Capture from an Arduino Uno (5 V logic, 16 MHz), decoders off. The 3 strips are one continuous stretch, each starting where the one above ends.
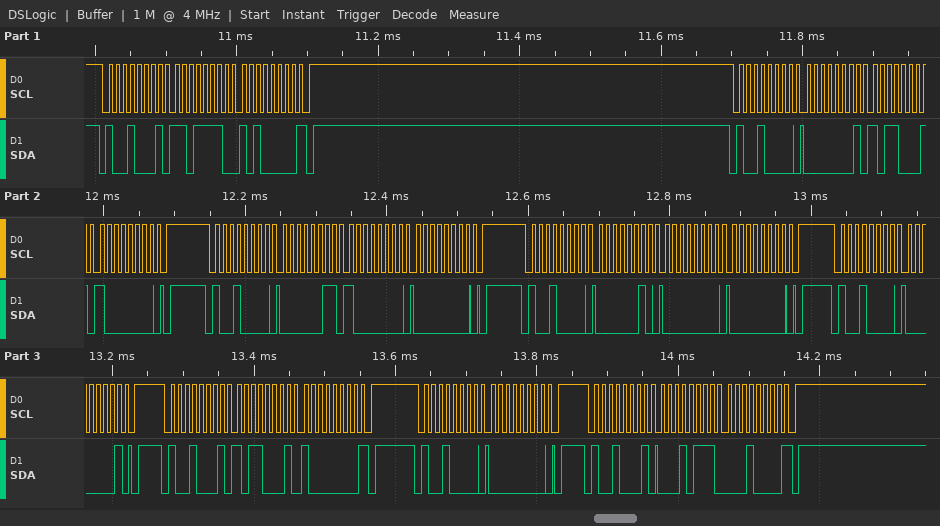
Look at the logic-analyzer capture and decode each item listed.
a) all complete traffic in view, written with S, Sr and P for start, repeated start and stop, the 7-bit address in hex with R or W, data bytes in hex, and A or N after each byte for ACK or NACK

S 48R A DE A A0 N P S 48W A 01 A B1 A 80 A P S 48W A 03 A 80 A 00 A P S 48W A 02 A 00 A 00 A P S 48W A 01 A P S 48R A B1 A 80 N P S 48W A 00 A P S 48R A 17 A 10 N P
